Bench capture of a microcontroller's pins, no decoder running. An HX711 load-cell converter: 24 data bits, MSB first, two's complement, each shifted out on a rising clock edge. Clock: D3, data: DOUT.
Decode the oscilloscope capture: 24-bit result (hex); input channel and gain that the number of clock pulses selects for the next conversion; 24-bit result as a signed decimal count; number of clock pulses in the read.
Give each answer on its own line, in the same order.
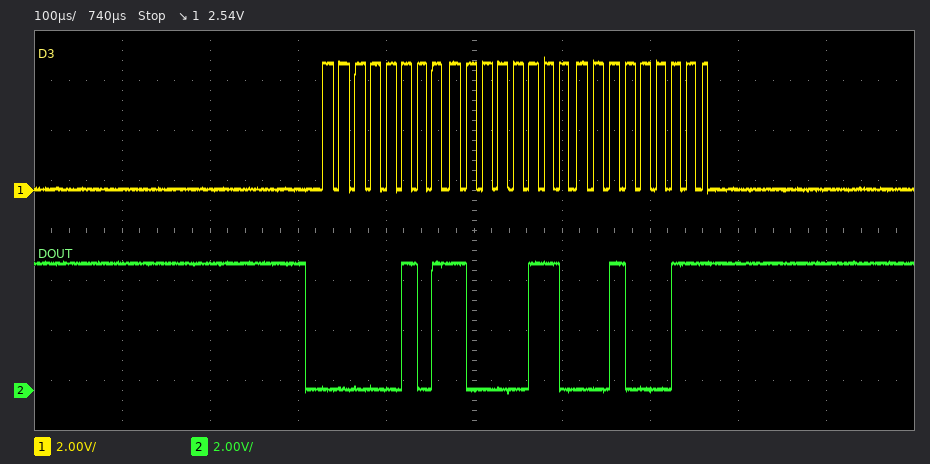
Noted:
0x058623
channel A, gain 128
362019
25
